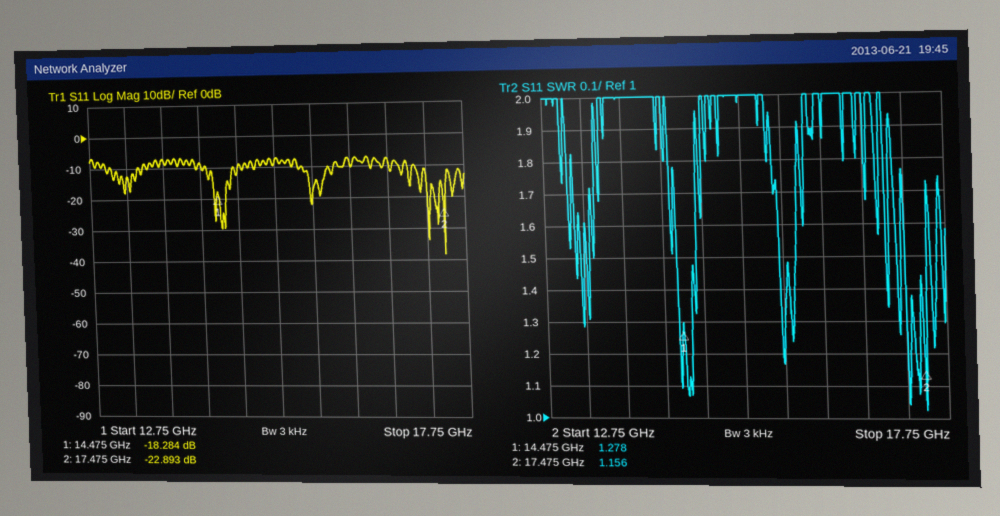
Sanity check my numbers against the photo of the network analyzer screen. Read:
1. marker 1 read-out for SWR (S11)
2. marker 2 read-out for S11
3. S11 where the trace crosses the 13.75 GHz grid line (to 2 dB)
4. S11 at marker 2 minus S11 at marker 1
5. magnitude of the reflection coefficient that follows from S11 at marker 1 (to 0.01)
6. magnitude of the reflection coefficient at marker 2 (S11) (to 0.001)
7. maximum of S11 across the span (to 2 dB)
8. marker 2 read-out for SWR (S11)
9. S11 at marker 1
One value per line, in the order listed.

1.278
-22.893 dB
-8 dB
-4.609 dB
0.12
0.072
-6 dB
1.156
-18.284 dB
